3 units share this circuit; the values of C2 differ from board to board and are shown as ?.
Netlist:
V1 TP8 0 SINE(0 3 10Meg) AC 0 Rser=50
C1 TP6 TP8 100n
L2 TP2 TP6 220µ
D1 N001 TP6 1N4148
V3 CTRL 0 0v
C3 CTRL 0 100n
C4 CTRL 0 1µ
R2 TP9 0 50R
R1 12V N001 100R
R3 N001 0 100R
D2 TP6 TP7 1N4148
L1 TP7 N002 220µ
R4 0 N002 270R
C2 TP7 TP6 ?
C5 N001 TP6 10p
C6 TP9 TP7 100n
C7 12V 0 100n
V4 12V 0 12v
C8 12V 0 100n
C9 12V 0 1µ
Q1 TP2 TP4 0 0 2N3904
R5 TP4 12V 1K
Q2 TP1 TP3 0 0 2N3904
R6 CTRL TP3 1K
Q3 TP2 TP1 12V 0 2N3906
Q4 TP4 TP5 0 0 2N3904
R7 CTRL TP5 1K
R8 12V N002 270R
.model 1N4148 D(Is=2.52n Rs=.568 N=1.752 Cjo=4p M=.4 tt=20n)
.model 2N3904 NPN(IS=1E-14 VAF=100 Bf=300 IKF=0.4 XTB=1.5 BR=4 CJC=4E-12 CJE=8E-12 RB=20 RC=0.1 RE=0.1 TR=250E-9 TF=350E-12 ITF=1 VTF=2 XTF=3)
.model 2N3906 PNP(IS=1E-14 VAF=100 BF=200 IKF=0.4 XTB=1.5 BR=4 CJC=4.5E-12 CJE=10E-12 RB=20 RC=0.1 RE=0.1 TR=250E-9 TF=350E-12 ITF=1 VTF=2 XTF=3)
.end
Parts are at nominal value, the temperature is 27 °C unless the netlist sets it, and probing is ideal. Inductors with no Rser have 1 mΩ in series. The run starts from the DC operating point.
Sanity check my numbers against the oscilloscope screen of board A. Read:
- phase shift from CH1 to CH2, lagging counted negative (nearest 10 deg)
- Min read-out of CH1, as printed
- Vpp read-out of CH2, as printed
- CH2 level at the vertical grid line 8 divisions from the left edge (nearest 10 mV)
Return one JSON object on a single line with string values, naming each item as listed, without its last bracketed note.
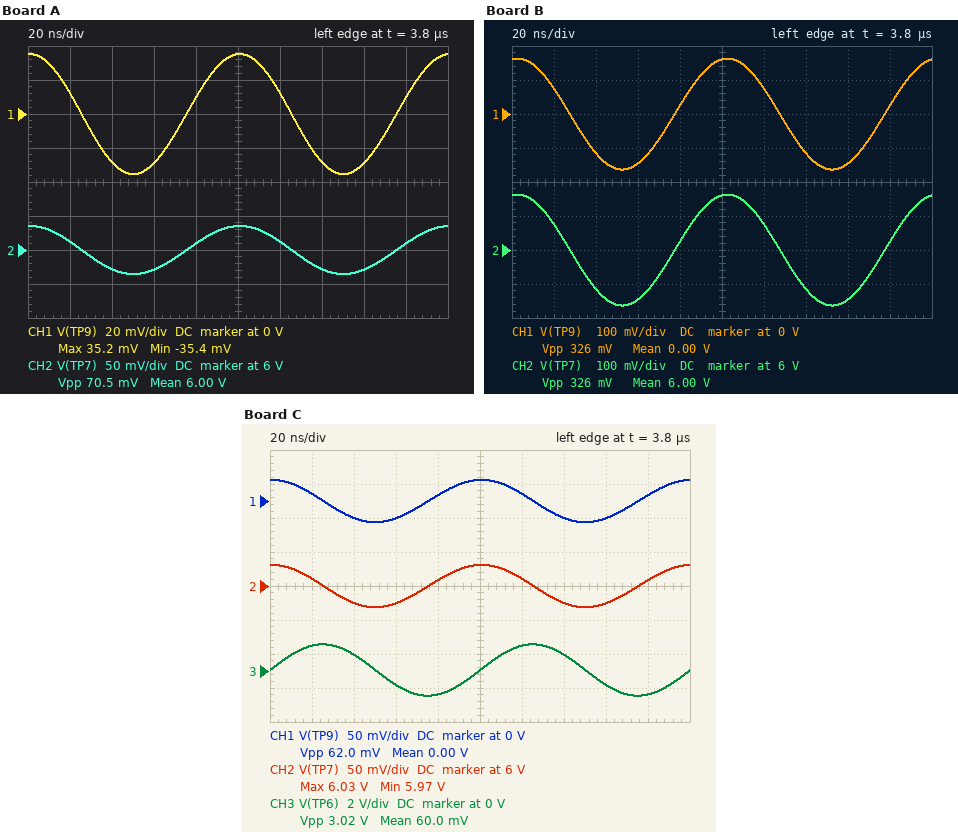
{"phase shift from CH1 to CH2, lagging counted negative": "0 deg", "Min read-out of CH1, as printed": "-35.4 mV", "Vpp read-out of CH2, as printed": "70.5 mV", "CH2 level at the vertical grid line 8 divisions from the left edge": "5.97 V"}
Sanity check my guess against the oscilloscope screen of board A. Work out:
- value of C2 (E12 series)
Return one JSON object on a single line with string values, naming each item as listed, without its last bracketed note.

{"value of C2": "5.6 pF"}
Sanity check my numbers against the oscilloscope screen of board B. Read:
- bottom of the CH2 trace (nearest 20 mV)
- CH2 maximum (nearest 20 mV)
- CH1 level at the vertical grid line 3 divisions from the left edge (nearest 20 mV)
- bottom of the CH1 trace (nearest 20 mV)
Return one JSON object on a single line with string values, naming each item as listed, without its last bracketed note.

{"bottom of the CH2 trace": "5.84 V", "CH2 maximum": "6.16 V", "CH1 level at the vertical grid line 3 divisions from the left edge": "-140 mV", "bottom of the CH1 trace": "-160 mV"}
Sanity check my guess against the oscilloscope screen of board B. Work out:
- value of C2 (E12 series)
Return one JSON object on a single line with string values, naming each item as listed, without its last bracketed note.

{"value of C2": "33 pF"}
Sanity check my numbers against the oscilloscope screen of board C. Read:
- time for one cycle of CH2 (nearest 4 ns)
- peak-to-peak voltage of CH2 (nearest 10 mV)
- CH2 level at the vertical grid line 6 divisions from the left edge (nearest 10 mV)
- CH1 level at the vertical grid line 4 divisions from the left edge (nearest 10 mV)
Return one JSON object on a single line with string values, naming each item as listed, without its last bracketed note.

{"time for one cycle of CH2": "100 ns", "peak-to-peak voltage of CH2": "60 mV", "CH2 level at the vertical grid line 6 divisions from the left edge": "6.01 V", "CH1 level at the vertical grid line 4 divisions from the left edge": "10 mV"}
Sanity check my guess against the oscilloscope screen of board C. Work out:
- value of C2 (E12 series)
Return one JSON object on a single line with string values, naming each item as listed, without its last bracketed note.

{"value of C2": "4.7 pF"}
